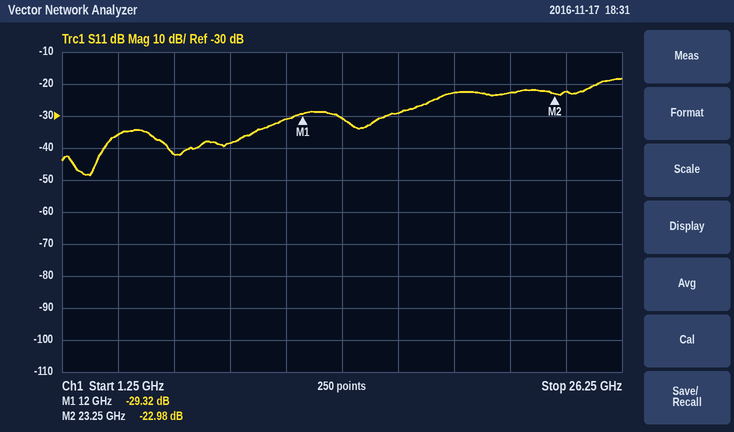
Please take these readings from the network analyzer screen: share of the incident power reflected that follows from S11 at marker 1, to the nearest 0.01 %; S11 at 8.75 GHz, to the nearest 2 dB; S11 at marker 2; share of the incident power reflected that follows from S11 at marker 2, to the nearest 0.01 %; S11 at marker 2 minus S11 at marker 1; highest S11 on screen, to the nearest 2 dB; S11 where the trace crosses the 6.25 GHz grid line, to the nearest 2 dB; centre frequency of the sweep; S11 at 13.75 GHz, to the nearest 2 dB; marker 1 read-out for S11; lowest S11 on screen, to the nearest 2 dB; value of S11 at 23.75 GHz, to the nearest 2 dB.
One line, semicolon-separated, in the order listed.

0.12 %; -38 dB; -22.98 dB; 0.50 %; 6.34 dB; -18 dB; -42 dB; 13.75 GHz; -30 dB; -29.32 dB; -48 dB; -22 dB
